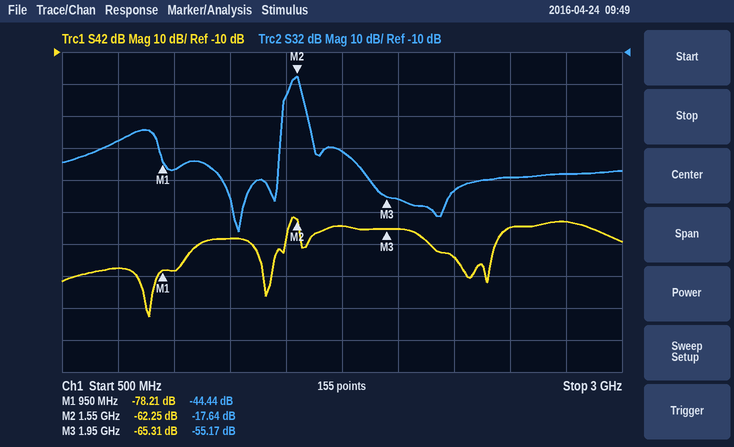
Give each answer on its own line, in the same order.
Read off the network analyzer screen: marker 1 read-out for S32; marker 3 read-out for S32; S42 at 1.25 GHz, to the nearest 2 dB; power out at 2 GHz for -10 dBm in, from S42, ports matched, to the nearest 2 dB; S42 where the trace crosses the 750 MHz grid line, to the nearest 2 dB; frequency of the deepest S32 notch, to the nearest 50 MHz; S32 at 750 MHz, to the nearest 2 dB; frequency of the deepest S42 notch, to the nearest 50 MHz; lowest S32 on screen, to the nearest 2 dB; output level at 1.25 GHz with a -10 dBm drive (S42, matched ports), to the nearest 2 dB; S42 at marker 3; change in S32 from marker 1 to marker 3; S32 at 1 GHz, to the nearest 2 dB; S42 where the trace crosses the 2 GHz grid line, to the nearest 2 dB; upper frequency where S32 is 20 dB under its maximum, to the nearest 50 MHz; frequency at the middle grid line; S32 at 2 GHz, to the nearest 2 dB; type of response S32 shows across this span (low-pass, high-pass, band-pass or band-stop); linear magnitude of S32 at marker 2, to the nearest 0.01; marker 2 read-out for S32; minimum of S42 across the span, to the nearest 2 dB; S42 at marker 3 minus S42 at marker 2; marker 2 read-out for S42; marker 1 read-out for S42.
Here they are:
-44.44 dB
-55.17 dB
-68 dB
-76 dBm
-78 dB
1.30 GHz
-38 dB
900 MHz
-66 dB
-78 dBm
-65.31 dB
-10.73 dB
-46 dB
-66 dB
1.60 GHz
1.75 GHz
-56 dB
band-pass
0.13
-17.64 dB
-92 dB
-3.06 dB
-62.25 dB
-78.21 dB
